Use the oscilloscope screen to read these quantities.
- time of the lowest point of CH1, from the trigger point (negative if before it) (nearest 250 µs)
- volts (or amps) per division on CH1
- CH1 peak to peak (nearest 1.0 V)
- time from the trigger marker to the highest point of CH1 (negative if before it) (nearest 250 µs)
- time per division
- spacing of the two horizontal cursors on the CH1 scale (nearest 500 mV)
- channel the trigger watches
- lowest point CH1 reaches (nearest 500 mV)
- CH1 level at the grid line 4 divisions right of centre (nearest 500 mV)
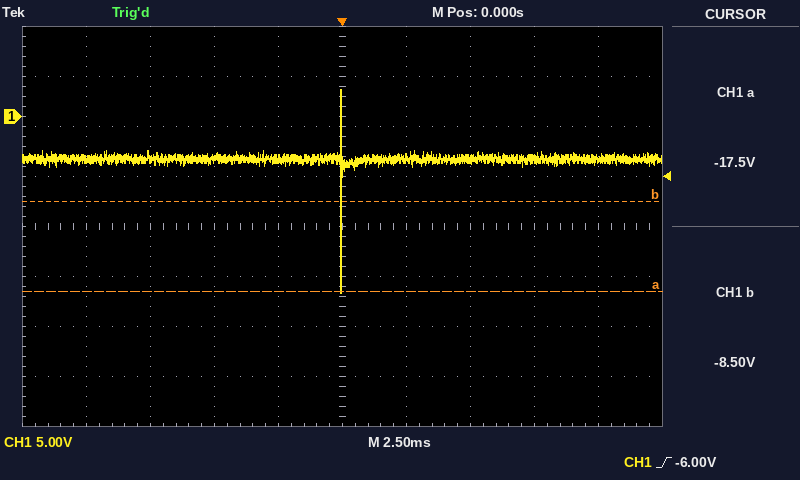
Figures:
0.00 ms
5 V
20.0 V
0.00 ms
2.5 ms
9.0 V
CH1
-17.5 V
-4.0 V
